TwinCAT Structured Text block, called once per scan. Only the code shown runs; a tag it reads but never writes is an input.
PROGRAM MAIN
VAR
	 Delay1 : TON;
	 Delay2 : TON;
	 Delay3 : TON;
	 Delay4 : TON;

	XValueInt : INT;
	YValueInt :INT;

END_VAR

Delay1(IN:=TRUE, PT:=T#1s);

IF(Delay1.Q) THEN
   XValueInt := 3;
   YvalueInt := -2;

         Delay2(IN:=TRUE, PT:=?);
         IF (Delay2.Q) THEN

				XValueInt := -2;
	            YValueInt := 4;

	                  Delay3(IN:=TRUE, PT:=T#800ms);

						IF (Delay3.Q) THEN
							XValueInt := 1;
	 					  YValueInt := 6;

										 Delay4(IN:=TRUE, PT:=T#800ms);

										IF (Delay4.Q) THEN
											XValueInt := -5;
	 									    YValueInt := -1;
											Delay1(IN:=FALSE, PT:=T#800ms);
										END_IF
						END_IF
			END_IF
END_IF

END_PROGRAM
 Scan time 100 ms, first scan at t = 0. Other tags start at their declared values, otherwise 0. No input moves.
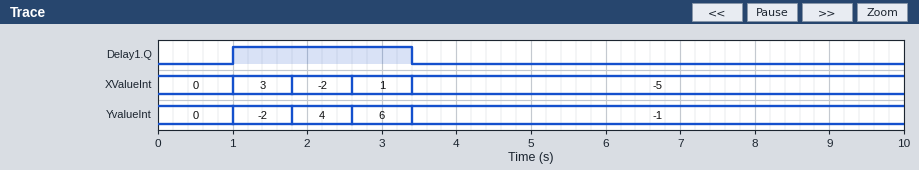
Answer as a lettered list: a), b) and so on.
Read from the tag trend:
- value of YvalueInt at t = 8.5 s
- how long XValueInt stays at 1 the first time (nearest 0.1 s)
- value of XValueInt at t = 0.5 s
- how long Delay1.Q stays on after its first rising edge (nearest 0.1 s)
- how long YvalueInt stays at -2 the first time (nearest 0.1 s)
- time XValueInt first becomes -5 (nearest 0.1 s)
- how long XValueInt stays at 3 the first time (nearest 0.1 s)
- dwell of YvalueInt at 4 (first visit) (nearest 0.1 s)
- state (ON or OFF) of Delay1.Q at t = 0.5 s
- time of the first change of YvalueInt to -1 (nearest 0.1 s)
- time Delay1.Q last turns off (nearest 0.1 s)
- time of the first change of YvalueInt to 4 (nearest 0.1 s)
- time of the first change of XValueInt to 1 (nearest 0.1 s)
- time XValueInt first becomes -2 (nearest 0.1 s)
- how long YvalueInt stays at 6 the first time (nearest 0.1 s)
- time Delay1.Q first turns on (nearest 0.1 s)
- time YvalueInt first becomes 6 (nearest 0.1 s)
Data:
a) -1
b) 0.8 s
c) 0
d) 2.4 s
e) 0.8 s
f) 3.4 s
g) 0.8 s
h) 0.8 s
i) OFF
j) 3.4 s
k) 3.4 s
l) 1.8 s
m) 2.6 s
n) 1.8 s
o) 0.8 s
p) 1.0 s
q) 2.6 s
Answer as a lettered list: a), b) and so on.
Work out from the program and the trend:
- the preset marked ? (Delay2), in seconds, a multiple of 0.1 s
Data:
a) 0.8 s
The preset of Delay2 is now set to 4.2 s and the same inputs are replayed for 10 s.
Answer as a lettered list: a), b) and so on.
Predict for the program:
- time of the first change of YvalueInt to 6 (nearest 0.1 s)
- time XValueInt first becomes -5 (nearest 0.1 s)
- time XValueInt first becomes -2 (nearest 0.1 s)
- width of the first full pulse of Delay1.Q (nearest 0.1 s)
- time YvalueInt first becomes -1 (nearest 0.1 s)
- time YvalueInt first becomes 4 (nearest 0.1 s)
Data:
a) 6.0 s
b) 6.8 s
c) 5.2 s
d) 5.8 s
e) 6.8 s
f) 5.2 s
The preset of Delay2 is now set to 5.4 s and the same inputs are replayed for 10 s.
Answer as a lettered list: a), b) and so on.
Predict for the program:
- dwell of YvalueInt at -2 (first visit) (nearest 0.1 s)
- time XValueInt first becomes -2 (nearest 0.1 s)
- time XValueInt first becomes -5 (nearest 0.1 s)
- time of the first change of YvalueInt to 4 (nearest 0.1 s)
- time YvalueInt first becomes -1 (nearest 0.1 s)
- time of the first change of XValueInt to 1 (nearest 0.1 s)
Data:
a) 5.4 s
b) 6.4 s
c) 8.0 s
d) 6.4 s
e) 8.0 s
f) 7.2 s
